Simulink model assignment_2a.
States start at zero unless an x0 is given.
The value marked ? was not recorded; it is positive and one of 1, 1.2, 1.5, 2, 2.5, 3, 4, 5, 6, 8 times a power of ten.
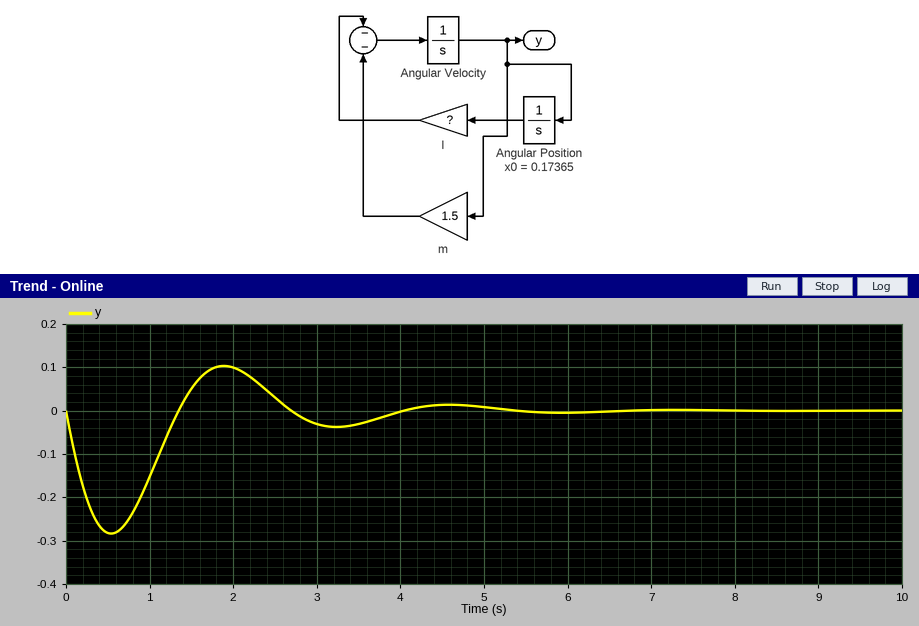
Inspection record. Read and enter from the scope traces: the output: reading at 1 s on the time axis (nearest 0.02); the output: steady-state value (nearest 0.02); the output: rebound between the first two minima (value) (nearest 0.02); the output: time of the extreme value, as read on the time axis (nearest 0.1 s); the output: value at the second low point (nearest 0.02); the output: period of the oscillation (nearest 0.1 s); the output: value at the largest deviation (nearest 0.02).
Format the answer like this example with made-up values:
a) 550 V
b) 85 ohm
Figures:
a) -0.16
b) 0.00
c) 0.10
d) 0.5 s
e) -0.04
f) 2.7 s
g) -0.28
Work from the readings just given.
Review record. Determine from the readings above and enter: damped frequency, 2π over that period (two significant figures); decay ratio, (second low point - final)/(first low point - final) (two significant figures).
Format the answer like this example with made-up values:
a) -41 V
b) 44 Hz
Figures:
a) 2.3 rad/s
b) 0.14
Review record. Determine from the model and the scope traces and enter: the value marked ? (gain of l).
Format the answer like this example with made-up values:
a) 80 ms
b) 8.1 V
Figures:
a) 6
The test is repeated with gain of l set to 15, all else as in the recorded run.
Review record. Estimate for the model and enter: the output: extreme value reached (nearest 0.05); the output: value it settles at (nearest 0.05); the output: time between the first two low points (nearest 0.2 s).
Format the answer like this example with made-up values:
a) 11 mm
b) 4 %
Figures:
a) -0.50
b) 0.00
c) 1.6 s
